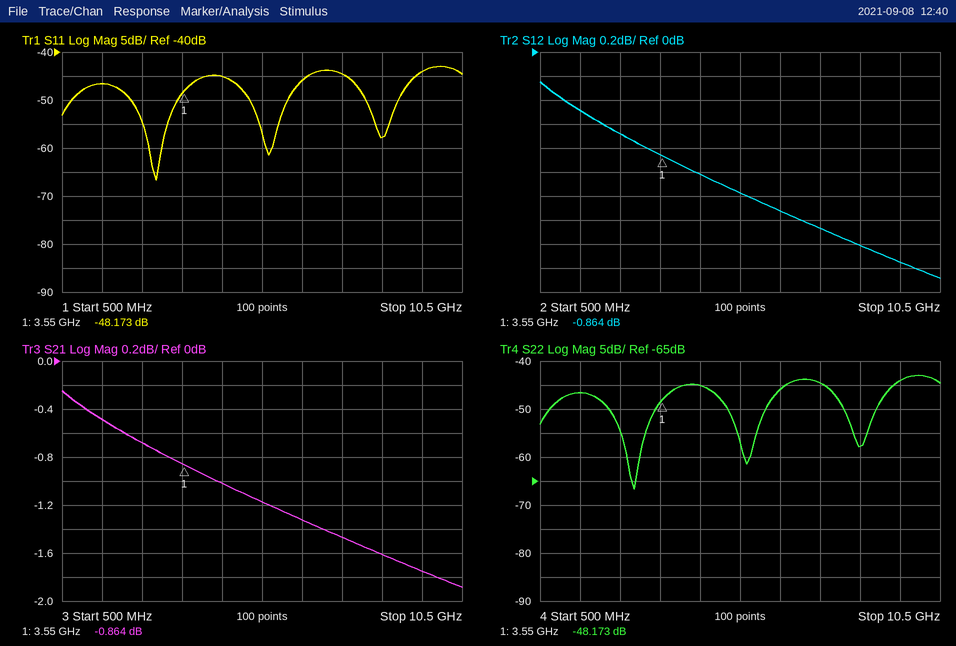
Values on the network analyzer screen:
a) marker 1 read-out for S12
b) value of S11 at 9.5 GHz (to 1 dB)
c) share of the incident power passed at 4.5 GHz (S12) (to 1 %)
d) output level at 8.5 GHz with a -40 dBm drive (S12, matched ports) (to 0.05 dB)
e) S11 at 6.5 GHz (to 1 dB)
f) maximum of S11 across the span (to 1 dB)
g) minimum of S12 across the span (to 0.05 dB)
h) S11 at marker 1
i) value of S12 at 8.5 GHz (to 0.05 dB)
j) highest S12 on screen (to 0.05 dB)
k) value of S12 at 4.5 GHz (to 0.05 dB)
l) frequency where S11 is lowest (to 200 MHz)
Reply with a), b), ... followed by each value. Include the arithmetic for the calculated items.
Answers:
a) -0.864 dB
b) -44 dB
c) 10^(-1/10) ≈ 79 %
d) -40 dBm + (-1.60 dB) = -41.60 dBm
e) -46 dB
f) -43 dB
g) -1.90 dB
h) -48.173 dB
i) -1.60 dB
j) -0.25 dB
k) -1.00 dB
l) 2.8 GHz
